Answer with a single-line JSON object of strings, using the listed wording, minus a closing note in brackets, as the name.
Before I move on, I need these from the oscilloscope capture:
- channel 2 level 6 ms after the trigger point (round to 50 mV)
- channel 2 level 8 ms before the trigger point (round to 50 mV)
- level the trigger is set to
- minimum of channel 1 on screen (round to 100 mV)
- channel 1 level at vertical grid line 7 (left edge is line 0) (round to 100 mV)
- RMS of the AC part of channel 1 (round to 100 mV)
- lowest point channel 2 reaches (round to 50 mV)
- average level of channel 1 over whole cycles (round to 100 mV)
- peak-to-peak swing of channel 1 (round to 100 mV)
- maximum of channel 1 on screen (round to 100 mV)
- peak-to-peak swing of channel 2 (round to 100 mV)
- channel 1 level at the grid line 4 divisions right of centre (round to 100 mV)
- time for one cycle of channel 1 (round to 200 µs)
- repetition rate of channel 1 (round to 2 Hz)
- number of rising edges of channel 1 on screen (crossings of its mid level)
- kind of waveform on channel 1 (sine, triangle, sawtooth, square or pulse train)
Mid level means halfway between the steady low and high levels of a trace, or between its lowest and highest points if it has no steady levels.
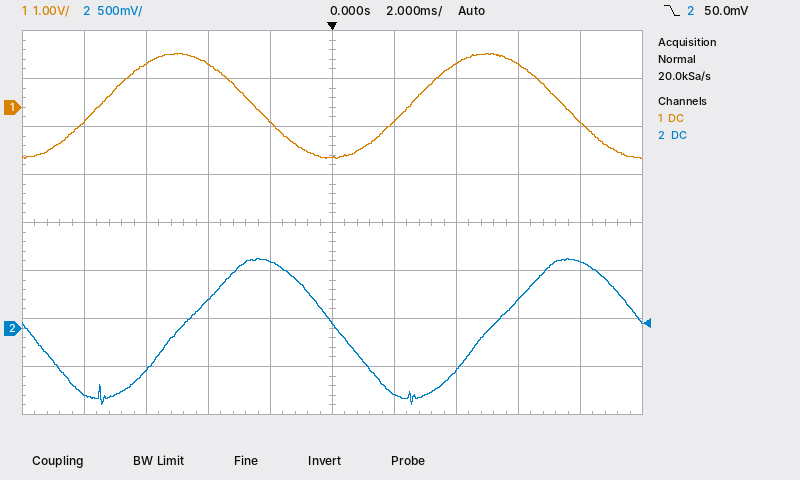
{"channel 2 level 6 ms after the trigger point": "300 mV", "channel 2 level 8 ms before the trigger point": "-700 mV", "level the trigger is set to": "50.0 mV", "minimum of channel 1 on screen": "-1.1 V", "channel 1 level at vertical grid line 7 (left edge is line 0)": "900 mV", "RMS of the AC part of channel 1": "800 mV", "lowest point channel 2 reaches": "-800 mV", "average level of channel 1 over whole cycles": "0.0 V", "peak-to-peak swing of channel 1": "2.2 V", "maximum of channel 1 on screen": "1.1 V", "peak-to-peak swing of channel 2": "1.50 V", "channel 1 level at the grid line 4 divisions right of centre": "-300 mV", "time for one cycle of channel 1": "10.0 ms", "repetition rate of channel 1": "100 Hz", "number of rising edges of channel 1 on screen": "2", "kind of waveform on channel 1": "sine"}
